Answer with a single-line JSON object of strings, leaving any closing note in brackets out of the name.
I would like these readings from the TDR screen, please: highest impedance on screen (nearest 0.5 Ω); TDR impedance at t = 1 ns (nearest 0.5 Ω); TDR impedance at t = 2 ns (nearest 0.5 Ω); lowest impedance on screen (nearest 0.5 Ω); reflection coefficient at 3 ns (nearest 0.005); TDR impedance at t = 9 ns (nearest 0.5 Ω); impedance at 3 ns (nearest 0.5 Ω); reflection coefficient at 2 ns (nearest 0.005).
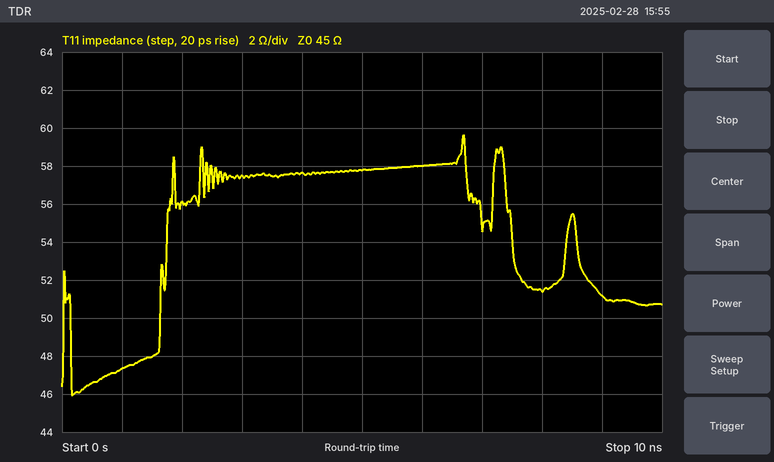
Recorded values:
{"highest impedance on screen": "59.5 Ω", "TDR impedance at t = 1 ns": "47.5 Ω", "TDR impedance at t = 2 ns": "56.0 Ω", "lowest impedance on screen": "46.0 Ω", "reflection coefficient at 3 ns": "+0.120", "TDR impedance at t = 9 ns": "51.0 Ω", "impedance at 3 ns": "57.5 Ω", "reflection coefficient at 2 ns": "+0.110"}
